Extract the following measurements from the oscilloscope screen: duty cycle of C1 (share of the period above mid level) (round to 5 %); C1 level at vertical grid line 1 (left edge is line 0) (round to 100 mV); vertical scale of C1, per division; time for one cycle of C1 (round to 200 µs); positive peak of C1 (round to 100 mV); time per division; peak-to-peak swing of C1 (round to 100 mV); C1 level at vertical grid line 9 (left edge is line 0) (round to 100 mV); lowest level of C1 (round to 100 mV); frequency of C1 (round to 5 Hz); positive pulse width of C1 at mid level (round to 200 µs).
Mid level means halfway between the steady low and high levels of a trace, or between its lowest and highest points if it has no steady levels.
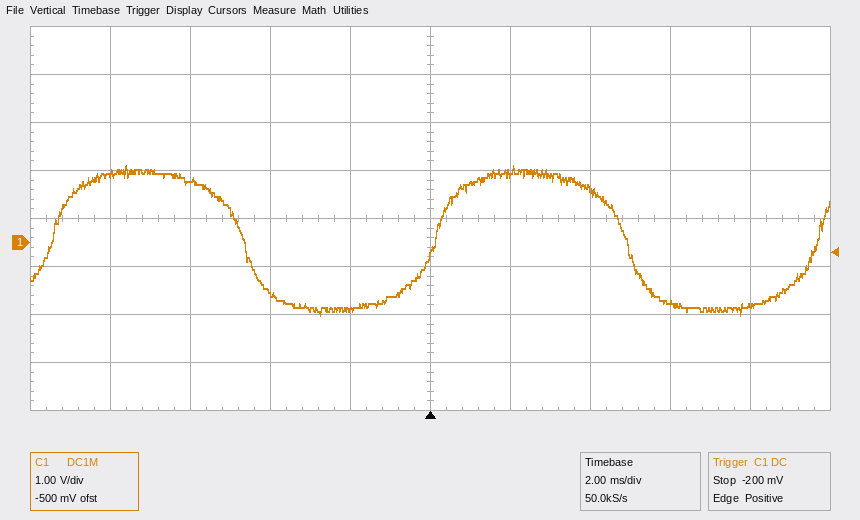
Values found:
50 %
1.4 V
1 V
9.6 ms
1.6 V
2 ms
3.1 V
-1.3 V
-1.5 V
105 Hz
4.8 ms
